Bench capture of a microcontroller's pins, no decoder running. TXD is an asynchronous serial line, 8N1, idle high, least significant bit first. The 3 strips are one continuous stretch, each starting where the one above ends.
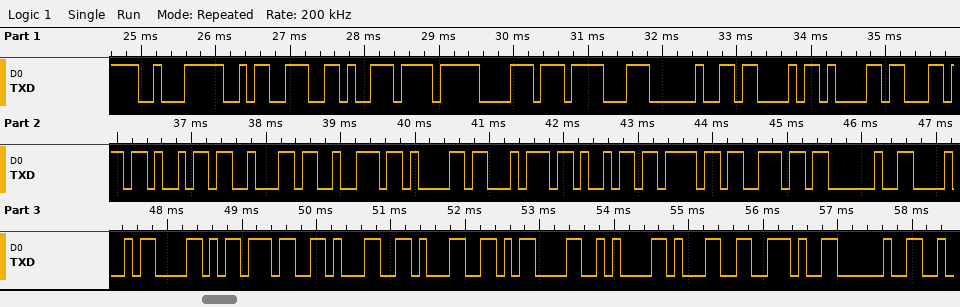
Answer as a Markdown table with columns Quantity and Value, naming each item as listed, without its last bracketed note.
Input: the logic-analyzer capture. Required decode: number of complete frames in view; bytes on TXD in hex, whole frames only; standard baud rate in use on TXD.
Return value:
| Quantity | Value |
|---|---|
| number of complete frames in view | 29 |
| bytes on TXD in hex, whole frames only | E2 9A 96 EF B8 8F 20 43 61 6C 69 62 72 61 74 69 6F 6E 20 48 58 37 31 31 0D 0A 31 2E 20 |
| standard baud rate in use on TXD | 9600 baud |
